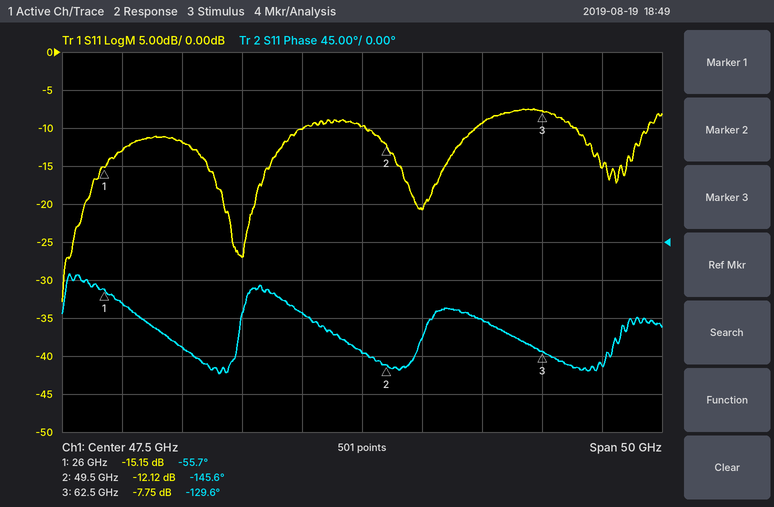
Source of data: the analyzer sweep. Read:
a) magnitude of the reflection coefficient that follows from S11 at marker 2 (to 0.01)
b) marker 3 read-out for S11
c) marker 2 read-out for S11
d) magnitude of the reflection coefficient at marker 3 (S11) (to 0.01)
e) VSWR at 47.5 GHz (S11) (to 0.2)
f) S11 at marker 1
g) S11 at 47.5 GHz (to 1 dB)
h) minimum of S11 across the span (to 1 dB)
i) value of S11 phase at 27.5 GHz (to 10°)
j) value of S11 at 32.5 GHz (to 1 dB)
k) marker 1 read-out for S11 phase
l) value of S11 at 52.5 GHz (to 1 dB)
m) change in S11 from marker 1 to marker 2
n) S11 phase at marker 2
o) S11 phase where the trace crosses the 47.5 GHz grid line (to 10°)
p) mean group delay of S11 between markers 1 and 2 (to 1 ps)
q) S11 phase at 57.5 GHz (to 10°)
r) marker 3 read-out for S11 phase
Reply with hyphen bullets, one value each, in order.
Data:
- 0.25
- -7.75 dB
- -12.12 dB
- 0.41
- 2.0
- -15.15 dB
- -10 dB
- -33 dB
- -70°
- -12 dB
- -55.7°
- -21 dB
- 3.03 dB
- -145.6°
- -130°
- 11 ps
- -90°
- -129.6°
